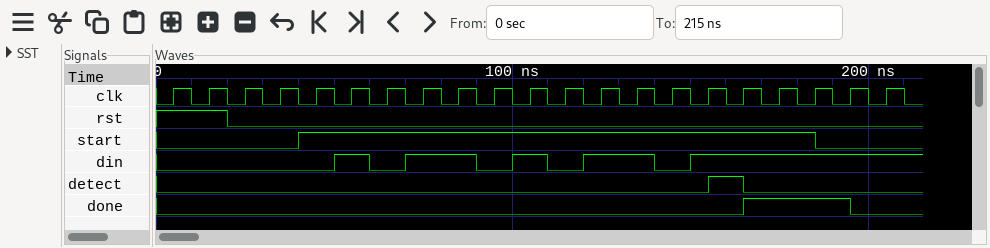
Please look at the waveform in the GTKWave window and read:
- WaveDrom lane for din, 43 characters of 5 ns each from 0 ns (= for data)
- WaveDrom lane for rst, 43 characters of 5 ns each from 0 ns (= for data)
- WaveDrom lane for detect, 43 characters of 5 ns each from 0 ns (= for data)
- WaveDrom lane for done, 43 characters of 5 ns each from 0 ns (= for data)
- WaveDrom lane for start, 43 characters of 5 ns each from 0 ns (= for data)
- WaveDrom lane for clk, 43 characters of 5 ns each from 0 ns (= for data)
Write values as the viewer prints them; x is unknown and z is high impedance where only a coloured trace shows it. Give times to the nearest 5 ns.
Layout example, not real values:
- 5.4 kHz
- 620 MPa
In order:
- {name: 'din', wave: '0.........1.0.1...0.1.0.1...0.1............'}
- {name: 'rst', wave: '1...0......................................'}
- {name: 'detect', wave: '0..............................1.0.........'}
- {name: 'done', wave: '0................................1.....0...'}
- {name: 'start', wave: '0.......1............................0.....'}
- {name: 'clk', wave: '0101010101010101010101010101010101010101010'}
